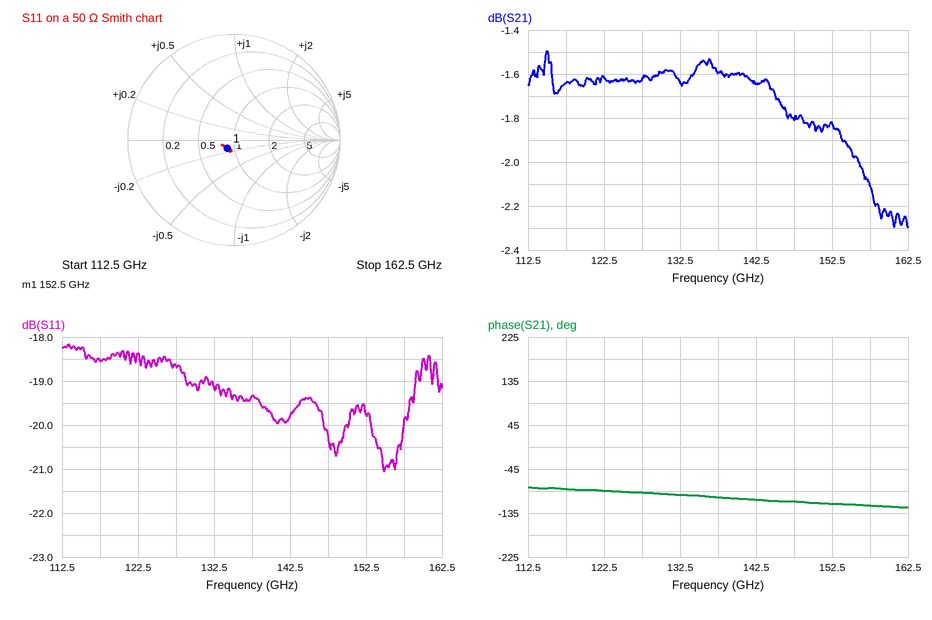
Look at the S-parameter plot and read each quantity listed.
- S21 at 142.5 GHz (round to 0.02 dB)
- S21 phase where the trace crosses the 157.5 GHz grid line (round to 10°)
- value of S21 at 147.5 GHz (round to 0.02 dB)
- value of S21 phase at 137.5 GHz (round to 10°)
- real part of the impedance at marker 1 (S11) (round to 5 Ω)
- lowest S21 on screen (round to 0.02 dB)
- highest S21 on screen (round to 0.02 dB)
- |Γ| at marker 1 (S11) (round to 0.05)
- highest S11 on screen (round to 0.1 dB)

-1.64 dB
-120°
-1.80 dB
-100°
45 Ω
-2.30 dB
-1.50 dB
0.10
-18.2 dB
